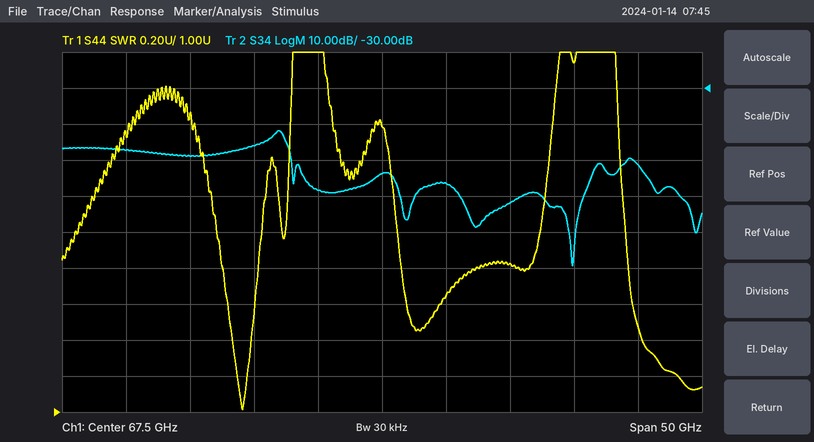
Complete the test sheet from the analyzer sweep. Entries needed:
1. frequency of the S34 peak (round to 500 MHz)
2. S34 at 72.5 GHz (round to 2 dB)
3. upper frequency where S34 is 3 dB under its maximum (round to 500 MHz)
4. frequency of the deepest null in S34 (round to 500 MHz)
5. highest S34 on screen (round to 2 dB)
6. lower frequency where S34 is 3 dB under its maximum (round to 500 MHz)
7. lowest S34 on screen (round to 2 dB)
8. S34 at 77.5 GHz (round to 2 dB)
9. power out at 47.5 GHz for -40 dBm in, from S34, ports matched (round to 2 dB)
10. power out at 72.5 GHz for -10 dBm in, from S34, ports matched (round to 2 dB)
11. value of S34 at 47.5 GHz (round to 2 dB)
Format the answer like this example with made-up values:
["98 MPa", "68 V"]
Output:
["59.5 GHz", "-56 dB", "60.0 GHz", "82.5 GHz", "-42 dB", "58.5 GHz", "-80 dB", "-62 dB", "-88 dBm", "-66 dBm", "-48 dB"]
